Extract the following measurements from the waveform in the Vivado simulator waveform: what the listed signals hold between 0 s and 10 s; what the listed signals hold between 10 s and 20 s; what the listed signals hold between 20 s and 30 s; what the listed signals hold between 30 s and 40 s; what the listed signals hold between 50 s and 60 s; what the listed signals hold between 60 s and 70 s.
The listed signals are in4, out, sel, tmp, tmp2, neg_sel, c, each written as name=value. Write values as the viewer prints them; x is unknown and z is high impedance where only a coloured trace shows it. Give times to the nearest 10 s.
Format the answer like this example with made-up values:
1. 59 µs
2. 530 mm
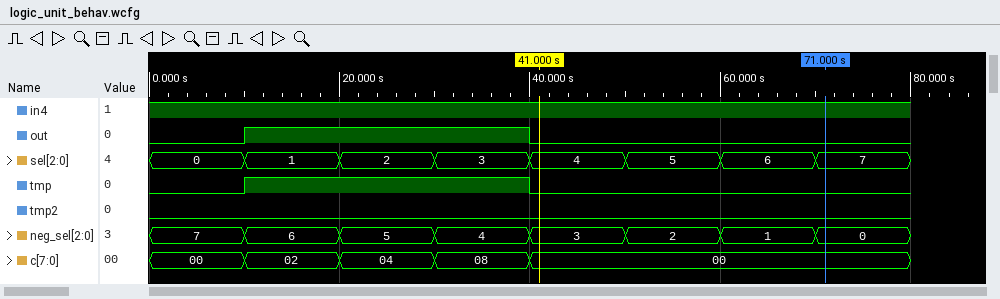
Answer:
1. in4=1, out=0, sel=0, tmp=0, tmp2=0, neg_sel=7, c=00
2. in4=1, out=1, sel=1, tmp=1, tmp2=0, neg_sel=6, c=02
3. in4=1, out=1, sel=2, tmp=1, tmp2=0, neg_sel=5, c=04
4. in4=1, out=1, sel=3, tmp=1, tmp2=0, neg_sel=4, c=08
5. in4=1, out=0, sel=5, tmp=0, tmp2=0, neg_sel=2, c=00
6. in4=1, out=0, sel=6, tmp=0, tmp2=0, neg_sel=1, c=00
